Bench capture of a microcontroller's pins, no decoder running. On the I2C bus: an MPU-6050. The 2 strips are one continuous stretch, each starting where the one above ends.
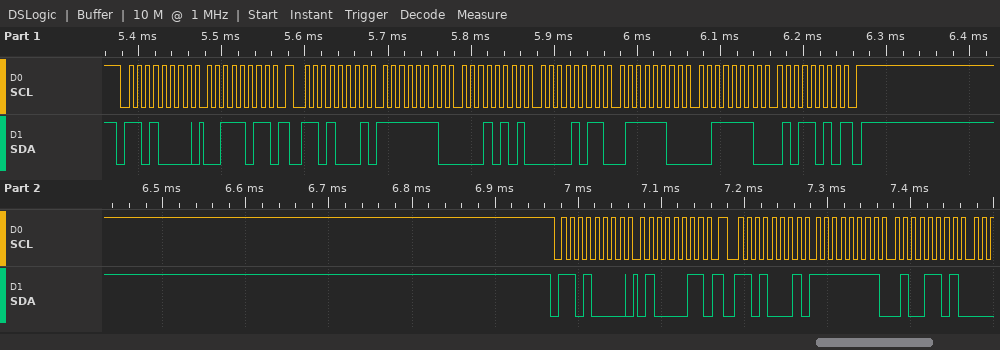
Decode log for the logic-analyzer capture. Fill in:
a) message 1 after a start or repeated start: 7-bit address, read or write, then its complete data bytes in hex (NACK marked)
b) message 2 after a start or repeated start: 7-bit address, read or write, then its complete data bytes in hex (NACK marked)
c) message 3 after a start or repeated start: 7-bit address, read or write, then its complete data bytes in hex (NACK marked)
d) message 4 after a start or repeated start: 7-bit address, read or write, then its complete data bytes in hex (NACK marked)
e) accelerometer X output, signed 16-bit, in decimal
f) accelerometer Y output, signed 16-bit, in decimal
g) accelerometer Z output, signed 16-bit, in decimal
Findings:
0x68 write: 3B
0x68 read: FE 15 0B 7C 3E 5A NACK
0x68 write: 43
0x68 read: FF 4D
-491
2940
15962
